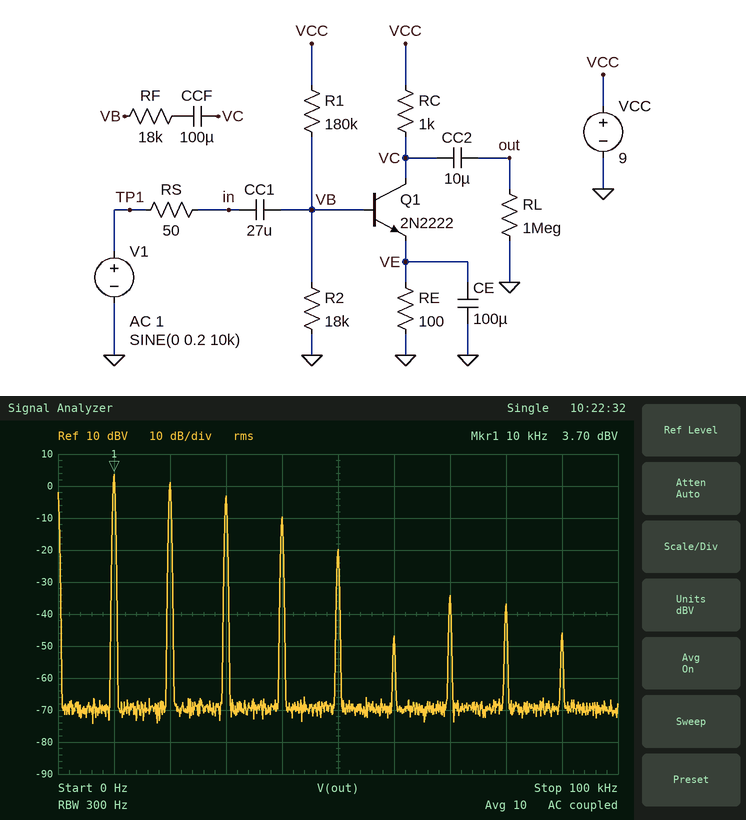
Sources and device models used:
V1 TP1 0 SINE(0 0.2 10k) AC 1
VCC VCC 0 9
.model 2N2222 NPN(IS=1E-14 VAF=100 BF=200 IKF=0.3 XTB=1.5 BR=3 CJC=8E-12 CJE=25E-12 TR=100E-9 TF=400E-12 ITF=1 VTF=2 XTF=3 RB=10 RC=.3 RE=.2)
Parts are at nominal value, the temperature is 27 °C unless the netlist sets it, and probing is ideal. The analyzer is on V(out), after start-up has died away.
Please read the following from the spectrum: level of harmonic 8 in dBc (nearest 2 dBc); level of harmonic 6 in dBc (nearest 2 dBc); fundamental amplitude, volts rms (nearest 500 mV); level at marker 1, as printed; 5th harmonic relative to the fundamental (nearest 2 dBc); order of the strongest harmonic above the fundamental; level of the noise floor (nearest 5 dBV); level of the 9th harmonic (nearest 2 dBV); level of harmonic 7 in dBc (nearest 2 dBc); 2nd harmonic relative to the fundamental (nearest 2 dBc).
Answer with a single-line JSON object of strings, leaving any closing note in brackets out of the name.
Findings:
{"level of harmonic 8 in dBc": "-40 dBc", "level of harmonic 6 in dBc": "-50 dBc", "fundamental amplitude, volts rms": "1.5 V", "level at marker 1, as printed": "3.70 dBV", "5th harmonic relative to the fundamental": "-24 dBc", "order of the strongest harmonic above the fundamental": "2", "level of the noise floor": "-70 dBV", "level of the 9th harmonic": "-46 dBV", "level of harmonic 7 in dBc": "-38 dBc", "2nd harmonic relative to the fundamental": "-2 dBc"}
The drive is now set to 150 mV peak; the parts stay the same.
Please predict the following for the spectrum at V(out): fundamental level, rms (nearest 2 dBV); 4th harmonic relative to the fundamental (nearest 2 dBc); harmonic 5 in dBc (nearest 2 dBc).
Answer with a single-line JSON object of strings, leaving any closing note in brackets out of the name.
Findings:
{"fundamental level, rms": "2 dBV", "4th harmonic relative to the fundamental": "-18 dBc", "harmonic 5 in dBc": "-32 dBc"}
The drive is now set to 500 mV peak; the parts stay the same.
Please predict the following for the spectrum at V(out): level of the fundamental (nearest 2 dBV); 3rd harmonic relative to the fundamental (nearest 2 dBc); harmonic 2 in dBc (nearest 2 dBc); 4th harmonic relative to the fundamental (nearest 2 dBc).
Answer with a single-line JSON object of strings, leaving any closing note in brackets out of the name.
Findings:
{"level of the fundamental": "6 dBV", "3rd harmonic relative to the fundamental": "-4 dBc", "harmonic 2 in dBc": "-2 dBc", "4th harmonic relative to the fundamental": "-8 dBc"}
